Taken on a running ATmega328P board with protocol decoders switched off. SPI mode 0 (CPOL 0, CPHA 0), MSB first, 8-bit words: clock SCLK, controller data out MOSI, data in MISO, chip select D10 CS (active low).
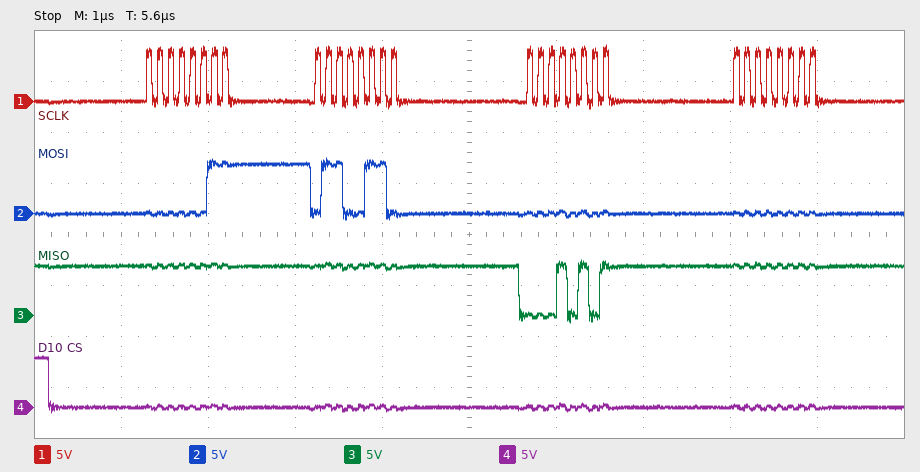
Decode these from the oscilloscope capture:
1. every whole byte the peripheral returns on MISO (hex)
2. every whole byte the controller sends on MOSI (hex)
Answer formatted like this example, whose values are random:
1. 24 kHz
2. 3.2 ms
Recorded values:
1. FF FF 15 FF
2. 03 66 00 00
